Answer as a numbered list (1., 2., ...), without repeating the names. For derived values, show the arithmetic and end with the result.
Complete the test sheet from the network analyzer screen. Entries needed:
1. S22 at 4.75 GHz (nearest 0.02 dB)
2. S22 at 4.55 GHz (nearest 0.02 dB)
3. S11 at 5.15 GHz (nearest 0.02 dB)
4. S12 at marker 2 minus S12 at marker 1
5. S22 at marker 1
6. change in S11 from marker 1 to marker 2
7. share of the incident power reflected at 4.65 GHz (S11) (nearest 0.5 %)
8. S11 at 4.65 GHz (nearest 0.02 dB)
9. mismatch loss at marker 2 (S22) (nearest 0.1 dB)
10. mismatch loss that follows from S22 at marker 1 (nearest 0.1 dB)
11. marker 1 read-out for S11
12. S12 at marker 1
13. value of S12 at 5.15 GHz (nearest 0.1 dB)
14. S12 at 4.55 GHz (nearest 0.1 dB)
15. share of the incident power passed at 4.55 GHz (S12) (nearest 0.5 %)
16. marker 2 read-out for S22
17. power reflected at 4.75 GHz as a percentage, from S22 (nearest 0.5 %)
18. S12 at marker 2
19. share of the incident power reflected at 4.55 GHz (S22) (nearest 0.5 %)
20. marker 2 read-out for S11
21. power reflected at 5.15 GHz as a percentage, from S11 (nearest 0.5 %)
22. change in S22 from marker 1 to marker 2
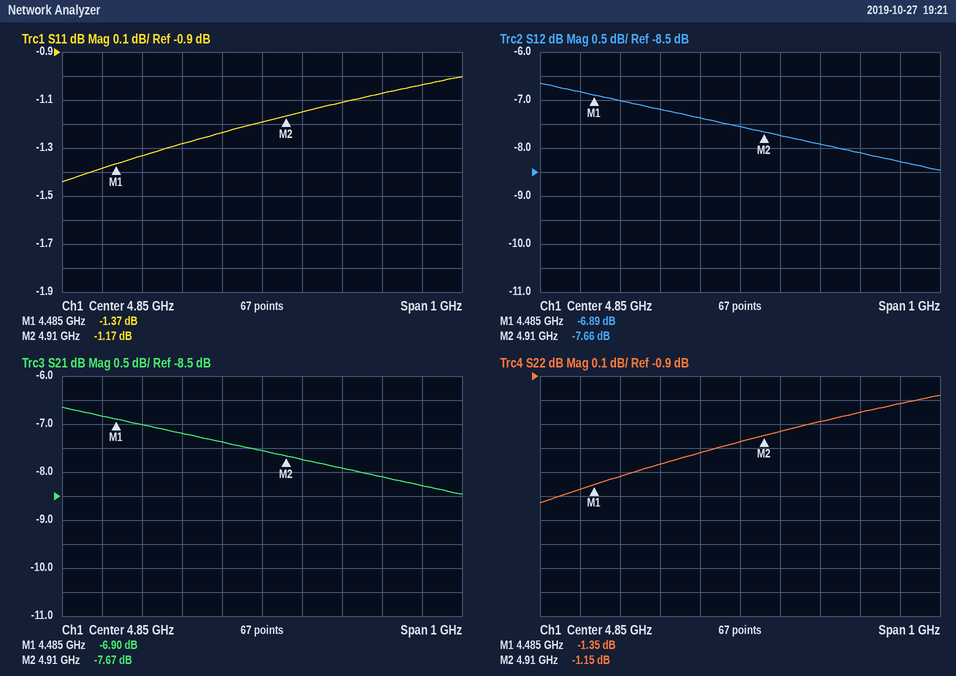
1. -1.22 dB
2. -1.32 dB
3. -1.08 dB
4. -7.66 − (-6.89) = -0.77 dB
5. -1.35 dB
6. -1.17 − (-1.37) = 0.20 dB
7. 10^(-1.28/10) ≈ 74.5 %
8. -1.28 dB
9. −10 log10(1 − 10^(-1.15/10)) ≈ 6.3 dB
10. −10 log10(1 − 10^(-1.35/10)) ≈ 5.7 dB
11. -1.37 dB
12. -6.89 dB
13. -8.1 dB
14. -7.0 dB
15. 10^(-7/10) ≈ 20.0 %
16. -1.15 dB
17. 10^(-1.22/10) ≈ 75.5 %
18. -7.66 dB
19. 10^(-1.32/10) ≈ 73.8 %, so 74.0 % to the nearest 0.5 %
20. -1.17 dB
21. 10^(-1.08/10) ≈ 78.0 %
22. -1.15 − (-1.35) = 0.20 dB
